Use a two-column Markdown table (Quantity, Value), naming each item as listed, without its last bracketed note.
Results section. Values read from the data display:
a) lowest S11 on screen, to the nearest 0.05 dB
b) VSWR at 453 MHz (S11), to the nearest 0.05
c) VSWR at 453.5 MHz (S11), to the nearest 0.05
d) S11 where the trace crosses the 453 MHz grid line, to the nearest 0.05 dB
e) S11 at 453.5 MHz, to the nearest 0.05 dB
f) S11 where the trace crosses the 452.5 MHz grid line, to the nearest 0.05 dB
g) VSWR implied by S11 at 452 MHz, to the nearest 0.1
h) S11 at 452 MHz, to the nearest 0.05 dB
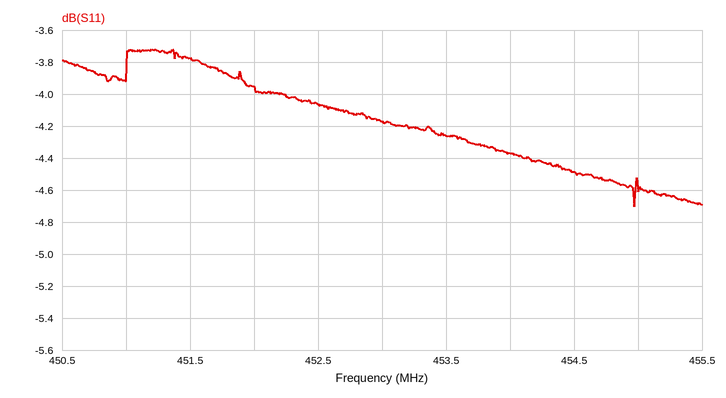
| Quantity | Value |
|---|---|
| lowest S11 on screen, to the nearest 0.05 dB | -4.70 dB |
| VSWR at 453 MHz (S11), to the nearest 0.05 | 4.25 |
| VSWR at 453.5 MHz (S11), to the nearest 0.05 | 4.15 |
| S11 where the trace crosses the 453 MHz grid line, to the nearest 0.05 dB | -4.15 dB |
| S11 at 453.5 MHz, to the nearest 0.05 dB | -4.25 dB |
| S11 where the trace crosses the 452.5 MHz grid line, to the nearest 0.05 dB | -4.05 dB |
| VSWR implied by S11 at 452 MHz, to the nearest 0.1 | 4.5 |
| S11 at 452 MHz, to the nearest 0.05 dB | -3.95 dB |
